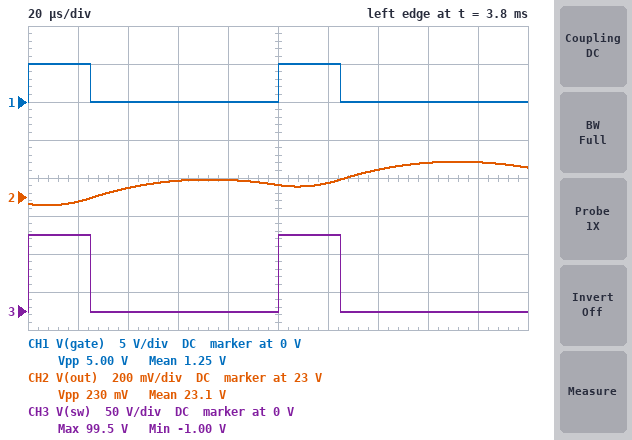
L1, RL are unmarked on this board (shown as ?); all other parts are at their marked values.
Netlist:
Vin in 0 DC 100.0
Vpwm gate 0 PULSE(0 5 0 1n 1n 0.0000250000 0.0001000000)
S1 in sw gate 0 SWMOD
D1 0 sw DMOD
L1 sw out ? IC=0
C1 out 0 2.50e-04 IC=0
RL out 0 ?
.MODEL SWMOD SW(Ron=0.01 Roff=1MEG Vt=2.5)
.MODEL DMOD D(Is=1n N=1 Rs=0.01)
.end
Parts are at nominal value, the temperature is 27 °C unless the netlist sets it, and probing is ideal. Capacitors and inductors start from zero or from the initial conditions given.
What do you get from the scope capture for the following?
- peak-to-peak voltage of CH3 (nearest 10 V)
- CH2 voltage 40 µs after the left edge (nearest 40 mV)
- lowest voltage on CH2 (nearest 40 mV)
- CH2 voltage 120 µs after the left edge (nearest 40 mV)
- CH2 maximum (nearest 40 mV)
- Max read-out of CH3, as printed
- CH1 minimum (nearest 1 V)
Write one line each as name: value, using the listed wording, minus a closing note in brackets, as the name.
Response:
peak-to-peak voltage of CH3: 100 V
CH2 voltage 40 µs after the left edge: 23.04 V
lowest voltage on CH2: 22.96 V
CH2 voltage 120 µs after the left edge: 23.08 V
CH2 maximum: 23.20 V
Max read-out of CH3, as printed: 99.5 V
CH1 minimum: 0 V
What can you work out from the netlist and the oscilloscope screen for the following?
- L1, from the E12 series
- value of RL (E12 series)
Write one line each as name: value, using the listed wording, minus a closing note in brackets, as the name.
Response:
L1, from the E12 series: 1.2 mH
value of RL: 0.82 Ω
